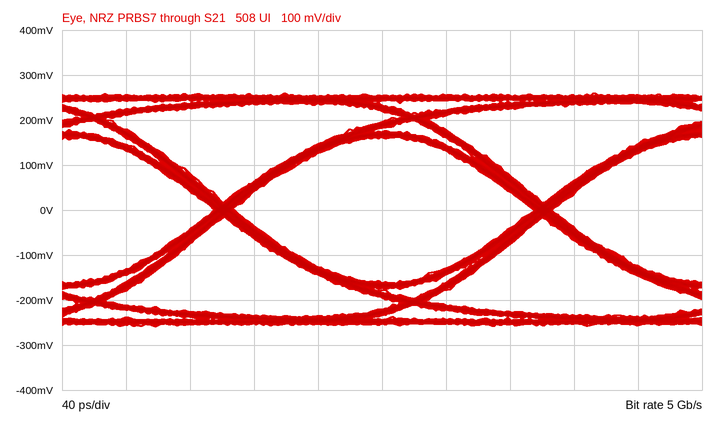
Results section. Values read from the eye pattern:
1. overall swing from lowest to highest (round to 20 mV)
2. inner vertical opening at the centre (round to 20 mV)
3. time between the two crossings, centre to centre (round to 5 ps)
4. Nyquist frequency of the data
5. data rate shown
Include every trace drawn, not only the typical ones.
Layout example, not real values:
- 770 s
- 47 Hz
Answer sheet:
- 520 mV
- 320 mV
- 200 ps
- 2.5 GHz
- 5 Gb/s
